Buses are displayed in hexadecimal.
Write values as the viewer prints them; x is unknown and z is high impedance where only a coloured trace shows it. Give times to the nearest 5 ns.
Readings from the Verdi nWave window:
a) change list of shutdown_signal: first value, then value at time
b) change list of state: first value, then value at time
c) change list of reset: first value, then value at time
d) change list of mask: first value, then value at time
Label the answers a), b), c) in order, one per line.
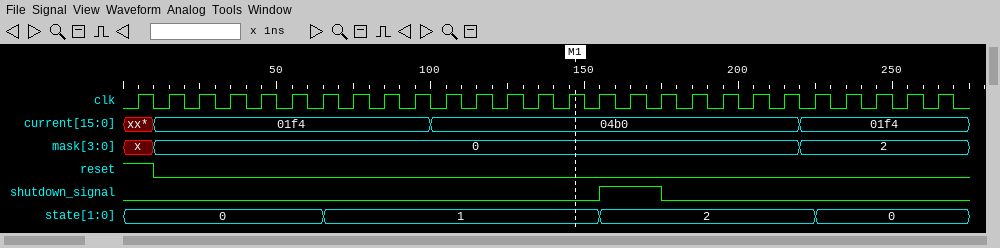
a) 0, 1 at 155 ns, 0 at 175 ns
b) 0, 1 at 65 ns, 2 at 155 ns, 0 at 225 ns
c) 1, 0 at 10 ns
d) x, 0 at 10 ns, 2 at 220 ns
